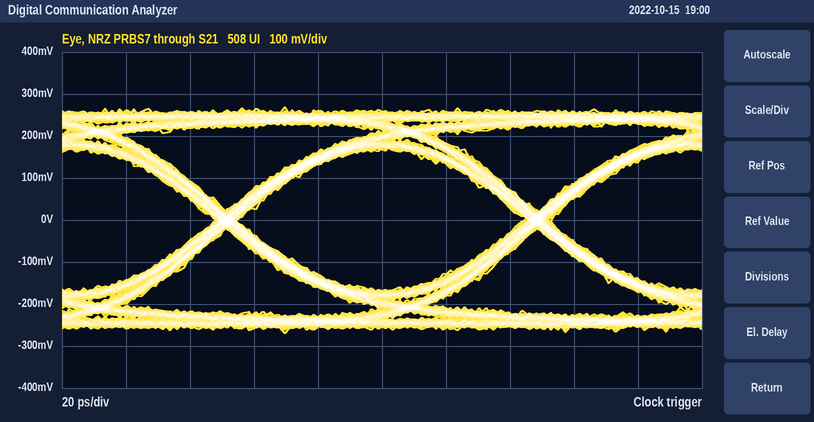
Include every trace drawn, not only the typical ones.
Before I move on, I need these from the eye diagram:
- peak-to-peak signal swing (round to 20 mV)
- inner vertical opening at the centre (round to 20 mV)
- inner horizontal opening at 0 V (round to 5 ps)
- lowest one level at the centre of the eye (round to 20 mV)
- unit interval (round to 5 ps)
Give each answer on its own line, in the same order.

540 mV
340 mV
90 ps
160 mV
95 ps
